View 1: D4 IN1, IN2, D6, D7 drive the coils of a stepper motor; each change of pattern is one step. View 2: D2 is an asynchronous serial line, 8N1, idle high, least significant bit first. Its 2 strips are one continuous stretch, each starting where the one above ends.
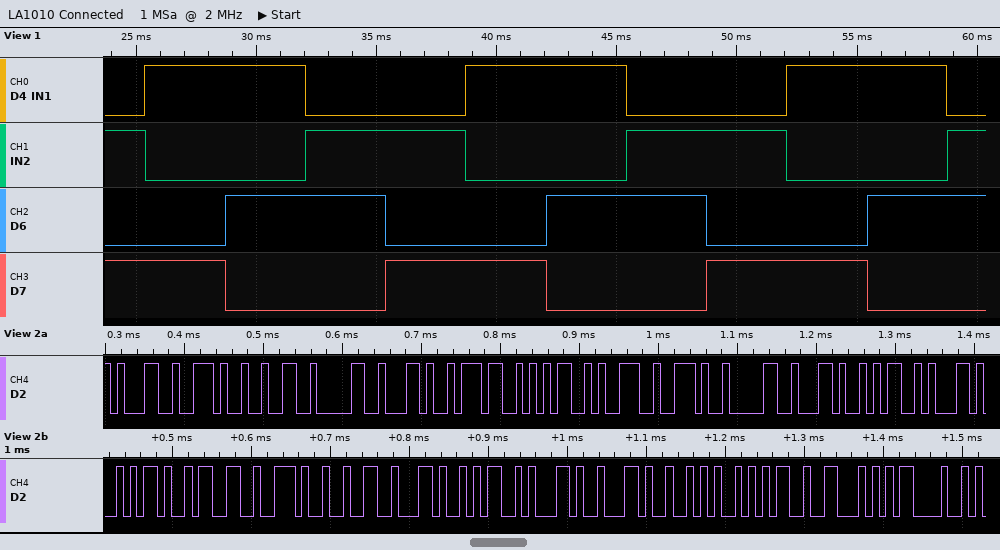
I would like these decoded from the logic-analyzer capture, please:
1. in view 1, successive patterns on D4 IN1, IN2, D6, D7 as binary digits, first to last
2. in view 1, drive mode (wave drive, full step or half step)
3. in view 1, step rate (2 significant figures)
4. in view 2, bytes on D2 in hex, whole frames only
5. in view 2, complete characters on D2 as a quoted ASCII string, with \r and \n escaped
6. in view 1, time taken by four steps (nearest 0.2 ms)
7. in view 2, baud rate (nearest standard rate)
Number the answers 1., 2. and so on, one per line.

1. 0101 1001 1010 0110 0101 1001 1010 0110 0101 1001 1010 0110
2. full step
3. 300 steps/s
4. 31 2E 32 30 2C 37 35 39 2E 30 2C 4D 2C 2D 33 2E 32 2C 4D 2C 2C 2A 35 46 0D
5. "1.20,759.0,M,-3.2,M,,*5F\r"
6. 13.4 ms
7. 115200 baud
